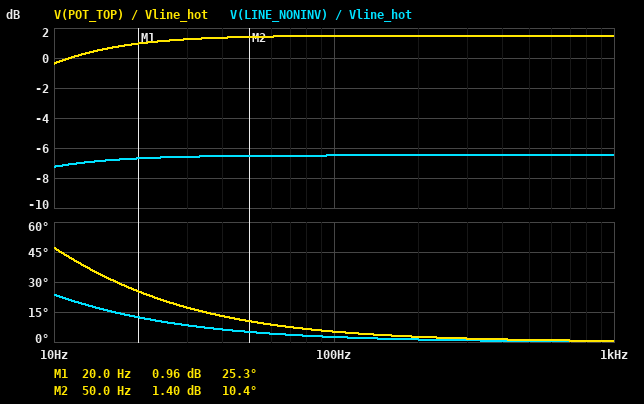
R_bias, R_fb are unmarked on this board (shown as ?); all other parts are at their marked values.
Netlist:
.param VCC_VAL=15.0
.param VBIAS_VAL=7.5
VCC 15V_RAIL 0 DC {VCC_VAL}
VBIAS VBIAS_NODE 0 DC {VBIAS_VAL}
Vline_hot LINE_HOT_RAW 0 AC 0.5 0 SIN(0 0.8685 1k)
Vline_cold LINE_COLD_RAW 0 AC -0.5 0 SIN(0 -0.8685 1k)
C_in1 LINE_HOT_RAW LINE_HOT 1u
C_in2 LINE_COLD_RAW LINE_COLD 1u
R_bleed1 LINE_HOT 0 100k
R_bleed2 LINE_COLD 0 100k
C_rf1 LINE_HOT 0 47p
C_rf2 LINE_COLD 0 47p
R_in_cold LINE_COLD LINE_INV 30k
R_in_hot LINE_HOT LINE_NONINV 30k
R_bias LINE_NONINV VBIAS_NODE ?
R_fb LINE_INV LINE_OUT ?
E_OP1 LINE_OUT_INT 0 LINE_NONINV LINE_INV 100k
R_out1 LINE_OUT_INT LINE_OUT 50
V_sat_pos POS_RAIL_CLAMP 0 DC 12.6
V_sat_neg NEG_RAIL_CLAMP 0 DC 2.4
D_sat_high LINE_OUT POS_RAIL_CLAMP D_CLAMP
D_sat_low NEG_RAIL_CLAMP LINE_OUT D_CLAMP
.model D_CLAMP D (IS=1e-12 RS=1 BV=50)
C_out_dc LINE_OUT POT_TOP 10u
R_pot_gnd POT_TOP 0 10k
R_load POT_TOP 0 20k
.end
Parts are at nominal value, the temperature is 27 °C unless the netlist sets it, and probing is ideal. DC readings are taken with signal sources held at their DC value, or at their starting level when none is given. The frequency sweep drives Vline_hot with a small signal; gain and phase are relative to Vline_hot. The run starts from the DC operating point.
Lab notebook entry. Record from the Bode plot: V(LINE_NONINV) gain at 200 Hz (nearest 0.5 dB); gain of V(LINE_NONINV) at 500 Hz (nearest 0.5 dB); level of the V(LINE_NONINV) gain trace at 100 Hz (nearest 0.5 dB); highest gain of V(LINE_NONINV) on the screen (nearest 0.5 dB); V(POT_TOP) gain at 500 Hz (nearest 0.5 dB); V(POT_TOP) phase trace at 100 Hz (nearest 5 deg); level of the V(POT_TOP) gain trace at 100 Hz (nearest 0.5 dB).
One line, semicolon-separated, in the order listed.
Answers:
-6.5 dB; -6.5 dB; -6.5 dB; -6.5 dB; 1.5 dB; 5 deg; 1.5 dB
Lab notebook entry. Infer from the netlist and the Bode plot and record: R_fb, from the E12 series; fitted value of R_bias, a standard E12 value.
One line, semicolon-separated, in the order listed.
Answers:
22 kΩ; 27 kΩ
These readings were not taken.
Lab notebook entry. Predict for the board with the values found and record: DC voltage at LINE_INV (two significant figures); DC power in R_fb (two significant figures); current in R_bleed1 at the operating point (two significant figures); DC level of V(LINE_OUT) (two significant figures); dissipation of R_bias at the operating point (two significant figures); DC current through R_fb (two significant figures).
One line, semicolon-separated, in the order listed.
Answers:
6.2 V; 50 µW; 48 µA; 7.3 V; 62 µW; 48 µA
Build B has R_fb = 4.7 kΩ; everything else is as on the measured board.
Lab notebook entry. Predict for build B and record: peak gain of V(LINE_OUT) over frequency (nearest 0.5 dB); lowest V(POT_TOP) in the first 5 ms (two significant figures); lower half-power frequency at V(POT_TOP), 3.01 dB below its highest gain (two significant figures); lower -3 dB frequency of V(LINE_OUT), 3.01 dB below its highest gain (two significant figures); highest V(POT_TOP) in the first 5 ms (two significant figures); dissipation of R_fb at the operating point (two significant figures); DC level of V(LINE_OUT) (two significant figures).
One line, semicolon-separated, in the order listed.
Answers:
-4.0 dB; -620 mV; 6.2 Hz; 5.3 Hz; 610 mV; 11 µW; 6.4 V
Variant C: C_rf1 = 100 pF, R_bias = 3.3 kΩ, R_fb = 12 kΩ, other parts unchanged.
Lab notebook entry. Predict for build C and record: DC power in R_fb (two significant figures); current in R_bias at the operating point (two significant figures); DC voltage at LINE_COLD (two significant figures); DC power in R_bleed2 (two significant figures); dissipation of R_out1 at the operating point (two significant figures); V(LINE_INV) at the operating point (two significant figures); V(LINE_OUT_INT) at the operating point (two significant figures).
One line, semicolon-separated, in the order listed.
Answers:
38 µW; 56 µA; 5.6 V; 320 µW; 160 nW; 7.3 V; 8.0 V
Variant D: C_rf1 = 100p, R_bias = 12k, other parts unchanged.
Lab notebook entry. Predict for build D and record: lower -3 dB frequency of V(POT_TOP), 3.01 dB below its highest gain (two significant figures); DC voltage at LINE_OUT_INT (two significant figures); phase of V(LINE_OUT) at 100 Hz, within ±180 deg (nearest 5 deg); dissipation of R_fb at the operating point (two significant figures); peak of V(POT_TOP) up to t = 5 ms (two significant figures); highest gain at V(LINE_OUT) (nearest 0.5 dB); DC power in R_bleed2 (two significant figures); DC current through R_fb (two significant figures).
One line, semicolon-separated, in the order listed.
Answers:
8.0 Hz; 8.0 V; 5 deg; 61 µW; 1.1 V; -1.5 dB; 280 µW; 53 µA
